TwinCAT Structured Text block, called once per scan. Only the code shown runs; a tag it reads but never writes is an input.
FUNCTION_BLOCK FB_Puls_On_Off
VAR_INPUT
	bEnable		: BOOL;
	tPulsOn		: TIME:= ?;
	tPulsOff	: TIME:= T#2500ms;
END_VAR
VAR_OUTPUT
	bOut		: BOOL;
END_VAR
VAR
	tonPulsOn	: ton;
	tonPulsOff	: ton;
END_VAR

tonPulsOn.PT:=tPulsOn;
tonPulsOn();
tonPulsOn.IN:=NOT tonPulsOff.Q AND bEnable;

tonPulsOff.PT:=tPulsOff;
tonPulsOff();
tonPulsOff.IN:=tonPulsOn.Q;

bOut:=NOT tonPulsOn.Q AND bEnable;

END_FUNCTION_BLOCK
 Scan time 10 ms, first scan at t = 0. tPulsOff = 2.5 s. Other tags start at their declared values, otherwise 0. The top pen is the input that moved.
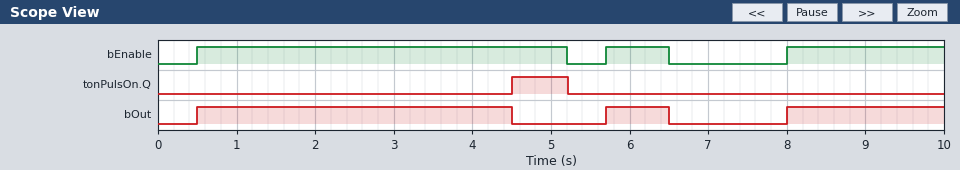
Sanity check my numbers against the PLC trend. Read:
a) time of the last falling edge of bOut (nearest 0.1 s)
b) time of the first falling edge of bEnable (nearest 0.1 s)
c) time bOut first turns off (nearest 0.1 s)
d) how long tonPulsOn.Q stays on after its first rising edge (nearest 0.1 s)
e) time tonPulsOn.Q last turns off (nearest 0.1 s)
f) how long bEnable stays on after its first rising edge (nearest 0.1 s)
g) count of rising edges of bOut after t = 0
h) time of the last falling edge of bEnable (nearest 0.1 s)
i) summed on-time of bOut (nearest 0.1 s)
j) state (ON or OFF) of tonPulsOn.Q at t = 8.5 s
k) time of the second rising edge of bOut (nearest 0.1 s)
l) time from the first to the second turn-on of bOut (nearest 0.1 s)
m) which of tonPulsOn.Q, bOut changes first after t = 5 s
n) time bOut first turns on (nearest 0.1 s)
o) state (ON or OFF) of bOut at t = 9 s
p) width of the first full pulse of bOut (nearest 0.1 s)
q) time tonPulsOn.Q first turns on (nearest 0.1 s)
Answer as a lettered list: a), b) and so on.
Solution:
a) 6.5 s
b) 5.2 s
c) 4.5 s
d) 0.7 s
e) 5.2 s
f) 4.7 s
g) 3
h) 6.5 s
i) 6.8 s
j) OFF
k) 5.7 s
l) 5.2 s
m) tonPulsOn.Q
n) 0.5 s
o) ON
p) 4.0 s
q) 4.5 s
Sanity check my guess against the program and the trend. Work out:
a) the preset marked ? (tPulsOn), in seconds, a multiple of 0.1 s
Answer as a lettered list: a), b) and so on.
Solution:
a) 4.0 s
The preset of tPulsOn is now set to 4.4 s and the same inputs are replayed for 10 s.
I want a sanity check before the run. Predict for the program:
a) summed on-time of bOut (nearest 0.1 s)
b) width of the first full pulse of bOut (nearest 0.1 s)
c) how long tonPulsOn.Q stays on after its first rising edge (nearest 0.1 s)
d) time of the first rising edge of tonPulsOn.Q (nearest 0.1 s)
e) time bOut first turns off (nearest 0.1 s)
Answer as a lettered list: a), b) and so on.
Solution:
a) 7.2 s
b) 4.4 s
c) 0.3 s
d) 4.9 s
e) 4.9 s
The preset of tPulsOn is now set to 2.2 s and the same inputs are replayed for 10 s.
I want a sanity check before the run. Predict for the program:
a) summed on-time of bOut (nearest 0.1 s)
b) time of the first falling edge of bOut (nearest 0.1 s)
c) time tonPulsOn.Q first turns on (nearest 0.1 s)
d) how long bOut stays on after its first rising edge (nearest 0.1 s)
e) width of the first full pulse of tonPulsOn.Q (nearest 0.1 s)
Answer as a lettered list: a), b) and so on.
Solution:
a) 5.0 s
b) 2.7 s
c) 2.7 s
d) 2.2 s
e) 2.5 s
